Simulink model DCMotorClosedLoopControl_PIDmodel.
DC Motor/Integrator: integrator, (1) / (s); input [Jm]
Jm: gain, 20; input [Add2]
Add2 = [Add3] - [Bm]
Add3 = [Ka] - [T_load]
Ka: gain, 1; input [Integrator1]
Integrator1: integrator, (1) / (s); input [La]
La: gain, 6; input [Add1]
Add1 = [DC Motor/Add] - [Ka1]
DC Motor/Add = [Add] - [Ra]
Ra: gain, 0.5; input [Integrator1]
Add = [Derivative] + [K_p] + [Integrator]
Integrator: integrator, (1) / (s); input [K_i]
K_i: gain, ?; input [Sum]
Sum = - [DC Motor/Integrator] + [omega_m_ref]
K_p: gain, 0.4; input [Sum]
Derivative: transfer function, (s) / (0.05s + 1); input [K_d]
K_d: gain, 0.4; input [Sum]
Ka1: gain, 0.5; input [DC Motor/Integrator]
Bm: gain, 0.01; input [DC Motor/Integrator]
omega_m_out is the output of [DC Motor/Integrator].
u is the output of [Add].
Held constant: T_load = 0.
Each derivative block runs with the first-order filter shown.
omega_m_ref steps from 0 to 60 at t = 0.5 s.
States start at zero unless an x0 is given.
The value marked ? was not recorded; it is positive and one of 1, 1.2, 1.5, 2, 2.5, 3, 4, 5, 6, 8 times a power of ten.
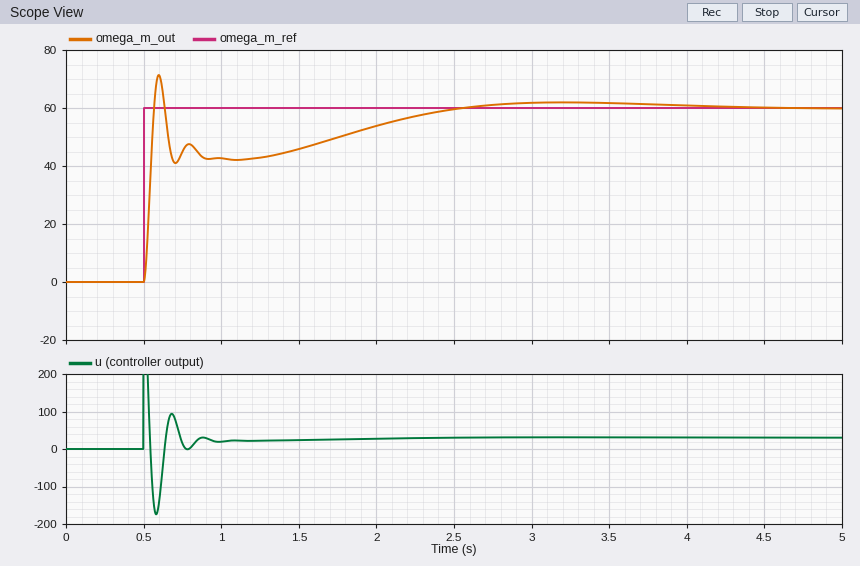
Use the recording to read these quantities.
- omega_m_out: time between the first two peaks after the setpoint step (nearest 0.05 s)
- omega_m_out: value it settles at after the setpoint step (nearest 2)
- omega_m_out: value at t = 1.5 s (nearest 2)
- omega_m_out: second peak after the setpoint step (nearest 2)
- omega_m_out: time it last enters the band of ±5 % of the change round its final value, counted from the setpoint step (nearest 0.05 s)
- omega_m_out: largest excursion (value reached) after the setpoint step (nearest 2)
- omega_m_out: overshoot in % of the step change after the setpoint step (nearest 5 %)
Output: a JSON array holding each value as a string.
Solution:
["0.20 s", "60", "46", "48", "1.75 s", "72", "20 %"]
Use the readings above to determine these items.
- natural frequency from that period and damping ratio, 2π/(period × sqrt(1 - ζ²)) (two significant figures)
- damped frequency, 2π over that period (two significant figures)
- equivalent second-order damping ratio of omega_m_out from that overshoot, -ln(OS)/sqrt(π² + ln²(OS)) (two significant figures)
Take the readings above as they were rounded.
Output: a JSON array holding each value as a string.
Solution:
["35 rad/s", "31 rad/s", "0.46"]
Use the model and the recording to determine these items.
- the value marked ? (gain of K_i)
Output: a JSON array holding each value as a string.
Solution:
["1.5"]
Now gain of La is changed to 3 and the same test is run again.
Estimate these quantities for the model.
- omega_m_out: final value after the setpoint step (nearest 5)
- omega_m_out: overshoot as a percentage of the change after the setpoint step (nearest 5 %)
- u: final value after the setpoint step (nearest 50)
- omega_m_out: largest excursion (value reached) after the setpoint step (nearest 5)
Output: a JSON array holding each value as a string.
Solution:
["60", "10 %", "50", "65"]
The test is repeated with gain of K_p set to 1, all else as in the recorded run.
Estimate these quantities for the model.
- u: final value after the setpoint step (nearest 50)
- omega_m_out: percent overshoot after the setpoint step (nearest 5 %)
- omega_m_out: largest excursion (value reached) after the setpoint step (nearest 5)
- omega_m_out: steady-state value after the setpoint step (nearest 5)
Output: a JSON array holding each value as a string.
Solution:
["50", "25 %", "75", "60"]
